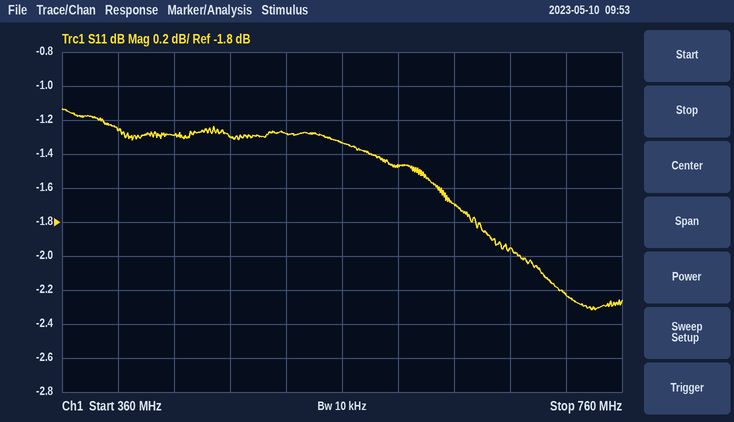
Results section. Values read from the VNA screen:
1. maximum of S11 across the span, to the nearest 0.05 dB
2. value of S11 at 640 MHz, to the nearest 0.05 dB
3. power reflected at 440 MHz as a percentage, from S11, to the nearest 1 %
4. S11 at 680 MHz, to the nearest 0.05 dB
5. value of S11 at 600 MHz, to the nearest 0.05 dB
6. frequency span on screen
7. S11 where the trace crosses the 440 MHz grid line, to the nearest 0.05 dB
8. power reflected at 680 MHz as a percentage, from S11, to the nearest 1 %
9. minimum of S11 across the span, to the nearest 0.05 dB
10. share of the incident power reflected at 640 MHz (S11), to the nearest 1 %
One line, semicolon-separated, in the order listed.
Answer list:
-1.15 dB; -1.70 dB; 74 %; -1.95 dB; -1.45 dB; 400 MHz; -1.30 dB; 64 %; -2.30 dB; 68 %
